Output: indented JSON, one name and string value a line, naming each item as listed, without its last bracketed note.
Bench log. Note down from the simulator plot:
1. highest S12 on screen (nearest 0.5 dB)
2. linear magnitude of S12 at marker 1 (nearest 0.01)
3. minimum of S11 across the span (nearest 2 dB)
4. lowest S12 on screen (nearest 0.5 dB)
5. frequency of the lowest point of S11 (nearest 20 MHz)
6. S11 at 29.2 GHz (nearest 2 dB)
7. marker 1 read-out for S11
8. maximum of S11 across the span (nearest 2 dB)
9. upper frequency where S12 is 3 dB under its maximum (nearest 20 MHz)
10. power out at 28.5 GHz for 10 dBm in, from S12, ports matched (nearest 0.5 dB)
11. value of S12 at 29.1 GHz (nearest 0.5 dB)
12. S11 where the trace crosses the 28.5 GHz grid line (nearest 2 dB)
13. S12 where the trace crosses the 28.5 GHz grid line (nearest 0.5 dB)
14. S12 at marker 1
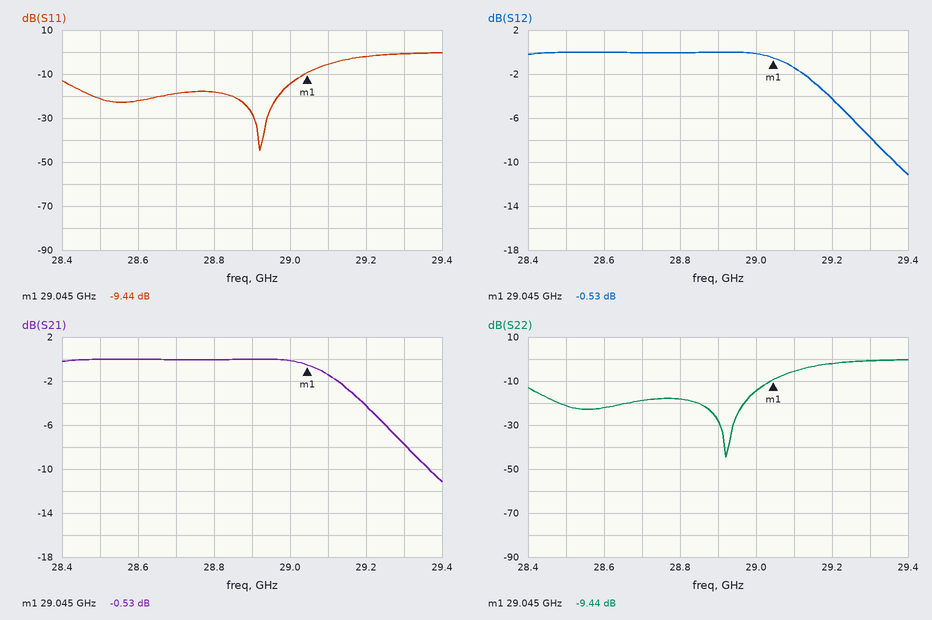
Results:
{
  "highest S12 on screen": "0.0 dB",
  "linear magnitude of S12 at marker 1": "0.94",
  "minimum of S11 across the span": "-44 dB",
  "lowest S12 on screen": "-11.0 dB",
  "frequency of the lowest point of S11": "28.92 GHz",
  "S11 at 29.2 GHz": "-2 dB",
  "marker 1 read-out for S11": "-9.44 dB",
  "maximum of S11 across the span": "0 dB",
  "upper frequency where S12 is 3 dB under its maximum": "29.16 GHz",
  "power out at 28.5 GHz for 10 dBm in, from S12, ports matched": "10.0 dBm",
  "value of S12 at 29.1 GHz": "-1.5 dB",
  "S11 where the trace crosses the 28.5 GHz grid line": "-22 dB",
  "S12 where the trace crosses the 28.5 GHz grid line": "0.0 dB",
  "S12 at marker 1": "-0.53 dB"
}
